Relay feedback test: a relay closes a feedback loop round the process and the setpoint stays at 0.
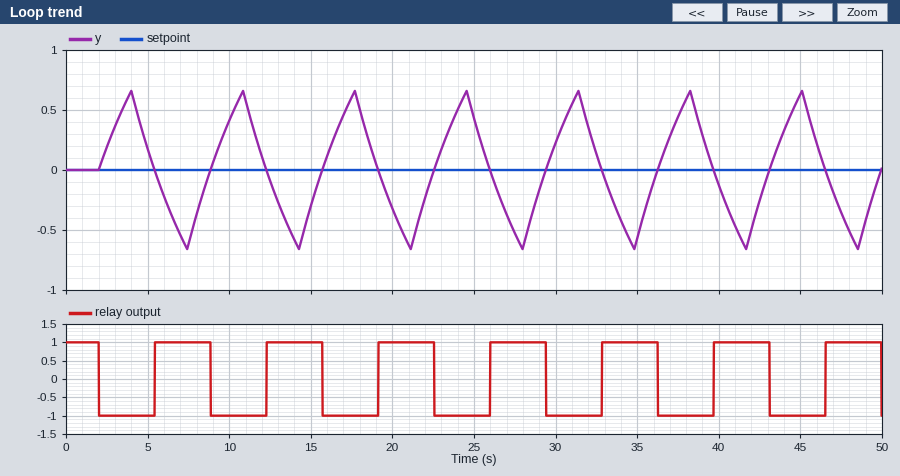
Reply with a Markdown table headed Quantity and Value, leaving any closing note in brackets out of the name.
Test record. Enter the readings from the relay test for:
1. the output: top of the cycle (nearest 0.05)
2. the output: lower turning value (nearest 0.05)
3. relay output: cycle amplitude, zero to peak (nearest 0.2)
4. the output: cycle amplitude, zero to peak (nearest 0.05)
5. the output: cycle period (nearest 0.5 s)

| Quantity | Value |
|---|---|
| the output: top of the cycle | 0.65 |
| the output: lower turning value | -0.65 |
| relay output: cycle amplitude, zero to peak | 1.0 |
| the output: cycle amplitude, zero to peak | 0.65 |
| the output: cycle period | 7.0 s |
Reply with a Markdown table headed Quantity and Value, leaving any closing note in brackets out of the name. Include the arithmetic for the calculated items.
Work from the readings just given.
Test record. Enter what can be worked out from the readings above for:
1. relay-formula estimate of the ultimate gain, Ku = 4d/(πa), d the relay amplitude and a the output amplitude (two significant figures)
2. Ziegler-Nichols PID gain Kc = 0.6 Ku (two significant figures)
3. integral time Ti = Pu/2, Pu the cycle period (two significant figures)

| Quantity | Value |
|---|---|
| relay-formula estimate of the ultimate gain, Ku = 4d/(πa), d the relay amplitude and a the output amplitude | 4 × 1 / (π × 0.65) = 2.0 |
| Ziegler-Nichols PID gain Kc = 0.6 Ku | 0.6 × 2 = 1.2 |
| integral time Ti = Pu/2, Pu the cycle period | 7 / 2 = 3.5 s |
